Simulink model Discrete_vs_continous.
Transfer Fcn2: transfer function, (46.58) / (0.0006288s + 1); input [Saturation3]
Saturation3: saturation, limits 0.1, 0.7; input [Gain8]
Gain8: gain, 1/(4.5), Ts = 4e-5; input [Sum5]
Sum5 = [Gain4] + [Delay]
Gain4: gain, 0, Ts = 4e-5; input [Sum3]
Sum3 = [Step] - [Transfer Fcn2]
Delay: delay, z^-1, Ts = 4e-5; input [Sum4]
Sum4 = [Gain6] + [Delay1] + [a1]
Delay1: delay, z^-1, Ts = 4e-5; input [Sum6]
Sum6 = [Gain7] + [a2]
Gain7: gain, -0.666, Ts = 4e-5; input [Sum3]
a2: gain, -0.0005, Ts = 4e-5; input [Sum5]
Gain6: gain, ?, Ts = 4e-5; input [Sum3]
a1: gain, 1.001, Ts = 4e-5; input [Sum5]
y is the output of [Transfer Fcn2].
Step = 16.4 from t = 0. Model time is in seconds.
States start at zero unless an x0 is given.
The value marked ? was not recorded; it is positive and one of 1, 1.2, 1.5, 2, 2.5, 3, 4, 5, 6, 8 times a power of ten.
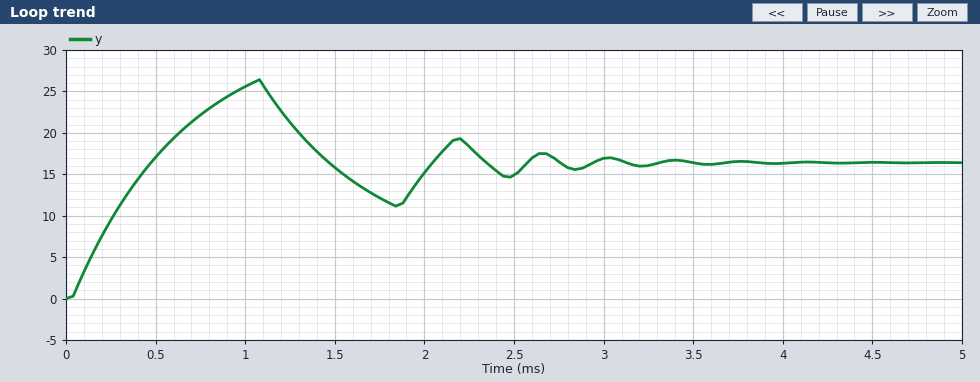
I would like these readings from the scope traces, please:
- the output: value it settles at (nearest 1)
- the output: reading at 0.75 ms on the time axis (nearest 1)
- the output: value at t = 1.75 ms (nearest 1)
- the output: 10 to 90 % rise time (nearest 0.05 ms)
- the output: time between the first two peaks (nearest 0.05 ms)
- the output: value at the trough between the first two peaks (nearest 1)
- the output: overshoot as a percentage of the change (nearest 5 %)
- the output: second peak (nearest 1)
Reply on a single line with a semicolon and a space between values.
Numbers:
16; 22; 12; 0.35 ms; 1.10 ms; 11; 60 %; 19
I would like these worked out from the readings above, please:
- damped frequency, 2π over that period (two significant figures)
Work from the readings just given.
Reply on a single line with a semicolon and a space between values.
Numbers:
5.7 rad/ms
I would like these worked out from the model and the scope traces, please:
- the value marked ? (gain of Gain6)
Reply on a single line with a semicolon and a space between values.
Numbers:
1
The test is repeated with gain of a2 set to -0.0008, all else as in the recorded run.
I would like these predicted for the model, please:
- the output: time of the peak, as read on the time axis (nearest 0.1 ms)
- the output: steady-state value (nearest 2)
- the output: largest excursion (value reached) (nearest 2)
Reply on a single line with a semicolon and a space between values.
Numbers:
1.1 ms; 16; 26
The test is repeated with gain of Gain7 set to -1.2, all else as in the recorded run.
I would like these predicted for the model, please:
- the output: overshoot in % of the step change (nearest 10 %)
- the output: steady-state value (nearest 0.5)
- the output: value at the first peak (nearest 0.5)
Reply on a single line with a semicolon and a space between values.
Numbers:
60 %; 4.5; 7.5
